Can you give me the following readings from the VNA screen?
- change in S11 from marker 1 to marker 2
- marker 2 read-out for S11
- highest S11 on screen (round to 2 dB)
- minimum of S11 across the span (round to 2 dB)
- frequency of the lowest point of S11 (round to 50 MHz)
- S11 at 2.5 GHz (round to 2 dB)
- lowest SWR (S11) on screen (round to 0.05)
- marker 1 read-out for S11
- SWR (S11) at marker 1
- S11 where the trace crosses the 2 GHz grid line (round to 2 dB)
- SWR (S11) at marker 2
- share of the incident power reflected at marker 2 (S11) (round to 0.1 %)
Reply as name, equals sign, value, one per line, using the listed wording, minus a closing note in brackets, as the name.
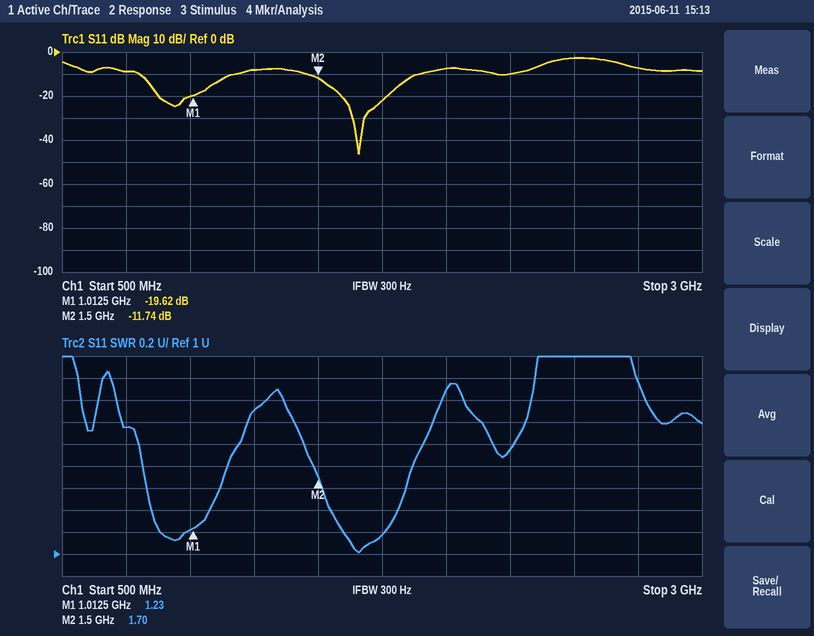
change in S11 from marker 1 to marker 2 = 7.88 dB
marker 2 read-out for S11 = -11.74 dB
highest S11 on screen = -2 dB
minimum of S11 across the span = -46 dB
frequency of the lowest point of S11 = 1.65 GHz
S11 at 2.5 GHz = -2 dB
lowest SWR (S11) on screen = 1.00
marker 1 read-out for S11 = -19.62 dB
SWR (S11) at marker 1 = 1.23
S11 where the trace crosses the 2 GHz grid line = -8 dB
SWR (S11) at marker 2 = 1.70
share of the incident power reflected at marker 2 (S11) = 6.7 %
